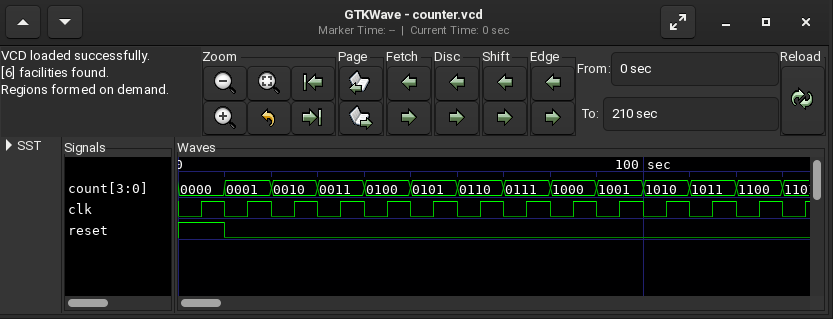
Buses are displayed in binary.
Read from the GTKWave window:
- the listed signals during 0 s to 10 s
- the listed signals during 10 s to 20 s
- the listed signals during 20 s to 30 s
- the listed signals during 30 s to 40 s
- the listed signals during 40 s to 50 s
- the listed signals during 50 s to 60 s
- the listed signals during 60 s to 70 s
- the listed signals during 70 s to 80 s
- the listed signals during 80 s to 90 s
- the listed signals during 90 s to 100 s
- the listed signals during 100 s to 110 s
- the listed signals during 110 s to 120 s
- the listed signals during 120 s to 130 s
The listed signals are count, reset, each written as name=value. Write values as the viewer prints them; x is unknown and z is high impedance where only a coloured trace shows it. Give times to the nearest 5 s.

count=0000, reset=1
count=0001, reset=0
count=0010, reset=0
count=0011, reset=0
count=0100, reset=0
count=0101, reset=0
count=0110, reset=0
count=0111, reset=0
count=1000, reset=0
count=1001, reset=0
count=1010, reset=0
count=1011, reset=0
count=1100, reset=0
